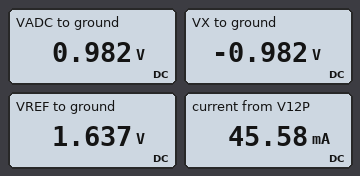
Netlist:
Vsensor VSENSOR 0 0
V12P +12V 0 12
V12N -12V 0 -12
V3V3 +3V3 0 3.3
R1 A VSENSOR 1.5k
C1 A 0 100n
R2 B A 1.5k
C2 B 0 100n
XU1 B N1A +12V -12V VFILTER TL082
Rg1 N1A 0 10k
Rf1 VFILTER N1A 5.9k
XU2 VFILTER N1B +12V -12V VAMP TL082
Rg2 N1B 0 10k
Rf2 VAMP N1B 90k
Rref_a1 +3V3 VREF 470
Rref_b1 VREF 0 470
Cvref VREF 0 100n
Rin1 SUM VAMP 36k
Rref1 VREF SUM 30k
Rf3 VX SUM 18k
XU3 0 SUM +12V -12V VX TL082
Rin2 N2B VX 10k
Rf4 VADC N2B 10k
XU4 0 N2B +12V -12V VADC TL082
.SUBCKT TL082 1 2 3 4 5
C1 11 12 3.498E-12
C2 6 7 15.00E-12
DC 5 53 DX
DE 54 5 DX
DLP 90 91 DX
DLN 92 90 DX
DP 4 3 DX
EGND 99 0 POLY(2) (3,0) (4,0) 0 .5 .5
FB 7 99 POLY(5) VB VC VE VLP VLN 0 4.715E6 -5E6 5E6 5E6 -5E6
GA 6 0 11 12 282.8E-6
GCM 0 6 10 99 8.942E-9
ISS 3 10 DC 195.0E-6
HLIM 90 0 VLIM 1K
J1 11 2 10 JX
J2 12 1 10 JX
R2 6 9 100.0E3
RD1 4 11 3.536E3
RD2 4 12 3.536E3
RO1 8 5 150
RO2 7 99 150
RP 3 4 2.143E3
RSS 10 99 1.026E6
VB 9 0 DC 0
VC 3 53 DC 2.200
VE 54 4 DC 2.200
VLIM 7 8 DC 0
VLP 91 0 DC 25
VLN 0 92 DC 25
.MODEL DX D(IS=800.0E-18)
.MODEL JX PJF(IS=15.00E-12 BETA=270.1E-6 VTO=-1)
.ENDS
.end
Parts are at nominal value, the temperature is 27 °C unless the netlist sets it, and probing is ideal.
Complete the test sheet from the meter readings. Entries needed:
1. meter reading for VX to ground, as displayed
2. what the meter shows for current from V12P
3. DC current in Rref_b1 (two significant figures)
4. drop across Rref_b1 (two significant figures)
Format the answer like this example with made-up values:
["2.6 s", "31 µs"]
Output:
["-0.982 V", "45.58 mA", "3.5 mA", "1.6 V"]
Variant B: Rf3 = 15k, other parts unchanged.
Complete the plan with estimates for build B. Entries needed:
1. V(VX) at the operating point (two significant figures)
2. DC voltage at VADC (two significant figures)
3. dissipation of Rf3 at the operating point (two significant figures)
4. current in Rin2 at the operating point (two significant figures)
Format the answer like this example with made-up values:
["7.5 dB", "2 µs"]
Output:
["-820 mV", "820 mV", "45 µW", "82 µA"]
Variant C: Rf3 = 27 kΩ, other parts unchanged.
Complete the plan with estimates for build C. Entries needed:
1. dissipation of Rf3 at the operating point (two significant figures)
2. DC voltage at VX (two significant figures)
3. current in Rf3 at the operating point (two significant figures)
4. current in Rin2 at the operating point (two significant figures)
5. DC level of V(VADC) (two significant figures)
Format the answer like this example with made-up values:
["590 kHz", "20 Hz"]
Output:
["80 µW", "-1.5 V", "55 µA", "150 µA", "1.5 V"]
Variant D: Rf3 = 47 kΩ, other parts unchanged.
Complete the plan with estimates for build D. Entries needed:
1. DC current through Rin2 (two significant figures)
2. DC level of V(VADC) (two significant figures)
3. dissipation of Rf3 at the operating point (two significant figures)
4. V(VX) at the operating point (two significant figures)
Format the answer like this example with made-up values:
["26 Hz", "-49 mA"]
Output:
["260 µA", "2.6 V", "140 µW", "-2.6 V"]
